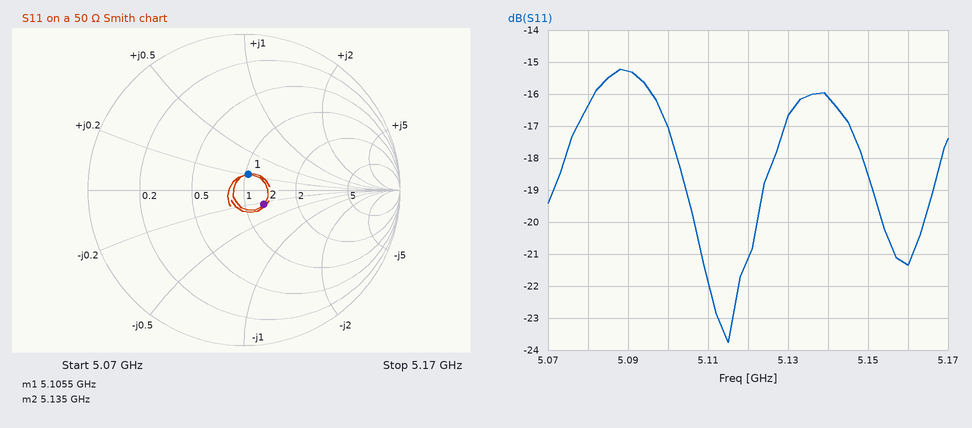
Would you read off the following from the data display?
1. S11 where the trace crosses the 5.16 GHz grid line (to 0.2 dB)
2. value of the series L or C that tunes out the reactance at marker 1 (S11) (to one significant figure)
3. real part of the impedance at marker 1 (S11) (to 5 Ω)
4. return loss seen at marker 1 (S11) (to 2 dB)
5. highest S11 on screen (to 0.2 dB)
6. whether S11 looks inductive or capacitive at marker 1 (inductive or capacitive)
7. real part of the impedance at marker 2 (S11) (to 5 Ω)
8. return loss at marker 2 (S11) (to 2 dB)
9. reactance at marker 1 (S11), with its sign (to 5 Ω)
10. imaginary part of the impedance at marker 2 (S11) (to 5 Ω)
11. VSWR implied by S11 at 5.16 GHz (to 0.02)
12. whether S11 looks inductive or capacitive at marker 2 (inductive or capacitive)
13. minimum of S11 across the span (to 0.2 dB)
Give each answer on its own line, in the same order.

-21.4 dB
3 pF
50 Ω
20 dB
-15.2 dB
inductive
65 Ω
16 dB
+10 Ω
-10 Ω
1.18
capacitive
-23.8 dB
